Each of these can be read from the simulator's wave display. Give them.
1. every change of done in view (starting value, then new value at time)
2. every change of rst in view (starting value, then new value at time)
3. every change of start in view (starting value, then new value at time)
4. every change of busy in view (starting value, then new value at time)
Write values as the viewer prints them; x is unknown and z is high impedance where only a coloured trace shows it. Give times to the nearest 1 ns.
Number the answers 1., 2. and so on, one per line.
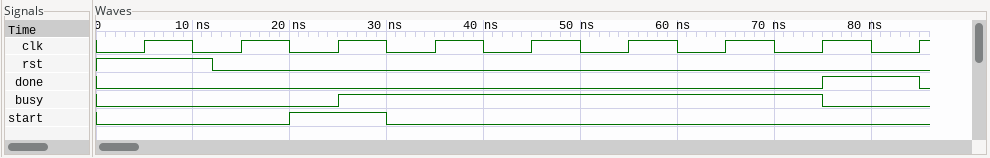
1. 0, 1 at 75 ns, 0 at 85 ns
2. 1, 0 at 12 ns
3. 0, 1 at 20 ns, 0 at 30 ns
4. 0, 1 at 25 ns, 0 at 75 ns
